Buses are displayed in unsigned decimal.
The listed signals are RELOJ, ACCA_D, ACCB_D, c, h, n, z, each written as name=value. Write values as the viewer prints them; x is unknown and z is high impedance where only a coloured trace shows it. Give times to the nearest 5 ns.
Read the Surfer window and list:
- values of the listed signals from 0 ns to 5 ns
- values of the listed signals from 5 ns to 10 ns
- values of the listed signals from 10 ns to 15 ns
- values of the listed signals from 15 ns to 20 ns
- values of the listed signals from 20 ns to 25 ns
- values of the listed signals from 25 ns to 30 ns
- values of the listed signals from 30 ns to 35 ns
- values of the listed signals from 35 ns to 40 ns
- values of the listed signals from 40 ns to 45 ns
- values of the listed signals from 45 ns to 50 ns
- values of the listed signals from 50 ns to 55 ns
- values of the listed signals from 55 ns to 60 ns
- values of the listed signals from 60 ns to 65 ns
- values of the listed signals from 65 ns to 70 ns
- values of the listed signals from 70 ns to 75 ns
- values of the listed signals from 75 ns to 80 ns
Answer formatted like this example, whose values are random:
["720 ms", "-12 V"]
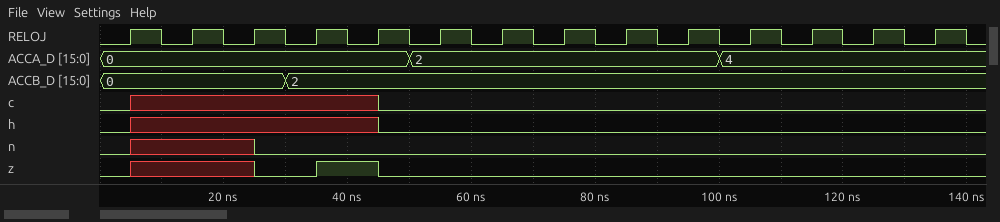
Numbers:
["RELOJ=0, ACCA_D=0, ACCB_D=0, c=0, h=0, n=0, z=0", "RELOJ=1, ACCA_D=0, ACCB_D=0, c=x, h=x, n=x, z=x", "RELOJ=0, ACCA_D=0, ACCB_D=0, c=x, h=x, n=x, z=x", "RELOJ=1, ACCA_D=0, ACCB_D=0, c=x, h=x, n=x, z=x", "RELOJ=0, ACCA_D=0, ACCB_D=0, c=x, h=x, n=x, z=x", "RELOJ=1, ACCA_D=0, ACCB_D=0, c=x, h=x, n=0, z=0", "RELOJ=0, ACCA_D=0, ACCB_D=2, c=x, h=x, n=0, z=0", "RELOJ=1, ACCA_D=0, ACCB_D=2, c=x, h=x, n=0, z=1", "RELOJ=0, ACCA_D=0, ACCB_D=2, c=x, h=x, n=0, z=1", "RELOJ=1, ACCA_D=0, ACCB_D=2, c=0, h=0, n=0, z=0", "RELOJ=0, ACCA_D=2, ACCB_D=2, c=0, h=0, n=0, z=0", "RELOJ=1, ACCA_D=2, ACCB_D=2, c=0, h=0, n=0, z=0", "RELOJ=0, ACCA_D=2, ACCB_D=2, c=0, h=0, n=0, z=0", "RELOJ=1, ACCA_D=2, ACCB_D=2, c=0, h=0, n=0, z=0", "RELOJ=0, ACCA_D=2, ACCB_D=2, c=0, h=0, n=0, z=0", "RELOJ=1, ACCA_D=2, ACCB_D=2, c=0, h=0, n=0, z=0"]
